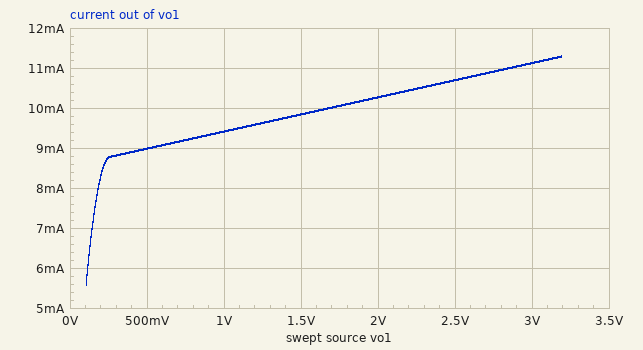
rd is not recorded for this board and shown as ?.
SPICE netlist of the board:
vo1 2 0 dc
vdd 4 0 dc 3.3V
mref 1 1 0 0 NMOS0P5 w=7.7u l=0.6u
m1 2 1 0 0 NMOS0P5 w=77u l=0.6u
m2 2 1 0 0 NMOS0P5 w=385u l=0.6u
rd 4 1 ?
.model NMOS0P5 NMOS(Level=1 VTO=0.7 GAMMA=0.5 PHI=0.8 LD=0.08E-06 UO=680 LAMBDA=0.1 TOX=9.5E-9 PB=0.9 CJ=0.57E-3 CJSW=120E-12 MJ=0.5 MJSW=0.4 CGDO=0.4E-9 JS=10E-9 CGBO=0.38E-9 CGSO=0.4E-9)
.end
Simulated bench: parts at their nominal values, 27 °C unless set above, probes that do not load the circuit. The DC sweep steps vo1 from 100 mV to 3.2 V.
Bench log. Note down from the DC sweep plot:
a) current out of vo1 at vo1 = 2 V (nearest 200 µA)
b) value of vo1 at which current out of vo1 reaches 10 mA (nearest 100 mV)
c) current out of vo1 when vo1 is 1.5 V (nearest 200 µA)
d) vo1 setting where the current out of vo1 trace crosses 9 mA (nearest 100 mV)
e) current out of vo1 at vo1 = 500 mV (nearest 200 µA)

10.2 mA
1.7 V
9.8 mA
500 mV
9.0 mA
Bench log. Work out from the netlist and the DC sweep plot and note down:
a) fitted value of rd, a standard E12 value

15 kΩ
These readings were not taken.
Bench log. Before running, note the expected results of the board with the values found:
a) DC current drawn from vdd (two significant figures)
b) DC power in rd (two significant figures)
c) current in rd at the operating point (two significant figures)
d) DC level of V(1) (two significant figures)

160 µA
370 µW
160 µA
960 mV
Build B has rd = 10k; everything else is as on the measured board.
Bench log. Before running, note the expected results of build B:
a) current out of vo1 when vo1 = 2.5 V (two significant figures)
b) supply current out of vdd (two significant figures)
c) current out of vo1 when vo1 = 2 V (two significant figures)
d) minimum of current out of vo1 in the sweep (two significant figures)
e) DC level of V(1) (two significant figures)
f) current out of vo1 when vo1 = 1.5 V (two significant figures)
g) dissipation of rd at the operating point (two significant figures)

16 mA
230 µA
15 mA
6.8 mA
1.0 V
14 mA
520 µW
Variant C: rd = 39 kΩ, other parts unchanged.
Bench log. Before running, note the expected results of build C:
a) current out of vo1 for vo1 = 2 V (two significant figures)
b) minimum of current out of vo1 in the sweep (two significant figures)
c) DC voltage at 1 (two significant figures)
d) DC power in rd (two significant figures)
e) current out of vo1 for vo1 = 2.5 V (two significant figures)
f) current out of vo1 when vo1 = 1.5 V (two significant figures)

4.1 mA
3.0 mA
860 mV
150 µW
4.3 mA
4.0 mA
